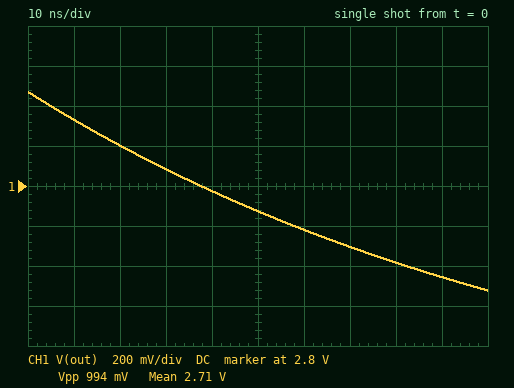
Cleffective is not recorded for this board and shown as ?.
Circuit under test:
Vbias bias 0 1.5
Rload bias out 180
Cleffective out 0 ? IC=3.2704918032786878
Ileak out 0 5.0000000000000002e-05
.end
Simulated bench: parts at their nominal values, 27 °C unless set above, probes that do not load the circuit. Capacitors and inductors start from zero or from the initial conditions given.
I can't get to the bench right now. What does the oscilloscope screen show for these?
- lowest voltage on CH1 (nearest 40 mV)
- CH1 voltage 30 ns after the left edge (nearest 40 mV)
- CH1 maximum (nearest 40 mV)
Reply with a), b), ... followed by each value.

a) 2.28 V
b) 2.88 V
c) 3.28 V
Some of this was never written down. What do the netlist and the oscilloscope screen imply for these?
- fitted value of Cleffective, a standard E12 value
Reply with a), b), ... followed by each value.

a) 680 pF
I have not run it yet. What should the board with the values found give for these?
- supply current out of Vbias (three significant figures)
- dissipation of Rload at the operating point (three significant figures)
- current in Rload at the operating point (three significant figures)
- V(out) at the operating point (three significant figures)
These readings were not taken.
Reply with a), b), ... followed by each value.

a) 50.0 µA
b) 450 nW
c) 50.0 µA
d) 1.49 V
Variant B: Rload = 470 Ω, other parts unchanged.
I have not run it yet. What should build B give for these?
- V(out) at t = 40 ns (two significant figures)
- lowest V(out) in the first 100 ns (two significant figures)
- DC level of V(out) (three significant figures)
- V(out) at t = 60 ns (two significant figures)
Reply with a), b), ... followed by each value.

a) 3.1 V
b) 2.8 V
c) 1.48 V
d) 3.0 V
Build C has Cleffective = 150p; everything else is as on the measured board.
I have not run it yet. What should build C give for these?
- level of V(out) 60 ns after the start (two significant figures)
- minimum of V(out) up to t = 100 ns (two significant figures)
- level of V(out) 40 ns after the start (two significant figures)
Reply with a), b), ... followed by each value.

a) 1.7 V
b) 1.5 V
c) 1.9 V
